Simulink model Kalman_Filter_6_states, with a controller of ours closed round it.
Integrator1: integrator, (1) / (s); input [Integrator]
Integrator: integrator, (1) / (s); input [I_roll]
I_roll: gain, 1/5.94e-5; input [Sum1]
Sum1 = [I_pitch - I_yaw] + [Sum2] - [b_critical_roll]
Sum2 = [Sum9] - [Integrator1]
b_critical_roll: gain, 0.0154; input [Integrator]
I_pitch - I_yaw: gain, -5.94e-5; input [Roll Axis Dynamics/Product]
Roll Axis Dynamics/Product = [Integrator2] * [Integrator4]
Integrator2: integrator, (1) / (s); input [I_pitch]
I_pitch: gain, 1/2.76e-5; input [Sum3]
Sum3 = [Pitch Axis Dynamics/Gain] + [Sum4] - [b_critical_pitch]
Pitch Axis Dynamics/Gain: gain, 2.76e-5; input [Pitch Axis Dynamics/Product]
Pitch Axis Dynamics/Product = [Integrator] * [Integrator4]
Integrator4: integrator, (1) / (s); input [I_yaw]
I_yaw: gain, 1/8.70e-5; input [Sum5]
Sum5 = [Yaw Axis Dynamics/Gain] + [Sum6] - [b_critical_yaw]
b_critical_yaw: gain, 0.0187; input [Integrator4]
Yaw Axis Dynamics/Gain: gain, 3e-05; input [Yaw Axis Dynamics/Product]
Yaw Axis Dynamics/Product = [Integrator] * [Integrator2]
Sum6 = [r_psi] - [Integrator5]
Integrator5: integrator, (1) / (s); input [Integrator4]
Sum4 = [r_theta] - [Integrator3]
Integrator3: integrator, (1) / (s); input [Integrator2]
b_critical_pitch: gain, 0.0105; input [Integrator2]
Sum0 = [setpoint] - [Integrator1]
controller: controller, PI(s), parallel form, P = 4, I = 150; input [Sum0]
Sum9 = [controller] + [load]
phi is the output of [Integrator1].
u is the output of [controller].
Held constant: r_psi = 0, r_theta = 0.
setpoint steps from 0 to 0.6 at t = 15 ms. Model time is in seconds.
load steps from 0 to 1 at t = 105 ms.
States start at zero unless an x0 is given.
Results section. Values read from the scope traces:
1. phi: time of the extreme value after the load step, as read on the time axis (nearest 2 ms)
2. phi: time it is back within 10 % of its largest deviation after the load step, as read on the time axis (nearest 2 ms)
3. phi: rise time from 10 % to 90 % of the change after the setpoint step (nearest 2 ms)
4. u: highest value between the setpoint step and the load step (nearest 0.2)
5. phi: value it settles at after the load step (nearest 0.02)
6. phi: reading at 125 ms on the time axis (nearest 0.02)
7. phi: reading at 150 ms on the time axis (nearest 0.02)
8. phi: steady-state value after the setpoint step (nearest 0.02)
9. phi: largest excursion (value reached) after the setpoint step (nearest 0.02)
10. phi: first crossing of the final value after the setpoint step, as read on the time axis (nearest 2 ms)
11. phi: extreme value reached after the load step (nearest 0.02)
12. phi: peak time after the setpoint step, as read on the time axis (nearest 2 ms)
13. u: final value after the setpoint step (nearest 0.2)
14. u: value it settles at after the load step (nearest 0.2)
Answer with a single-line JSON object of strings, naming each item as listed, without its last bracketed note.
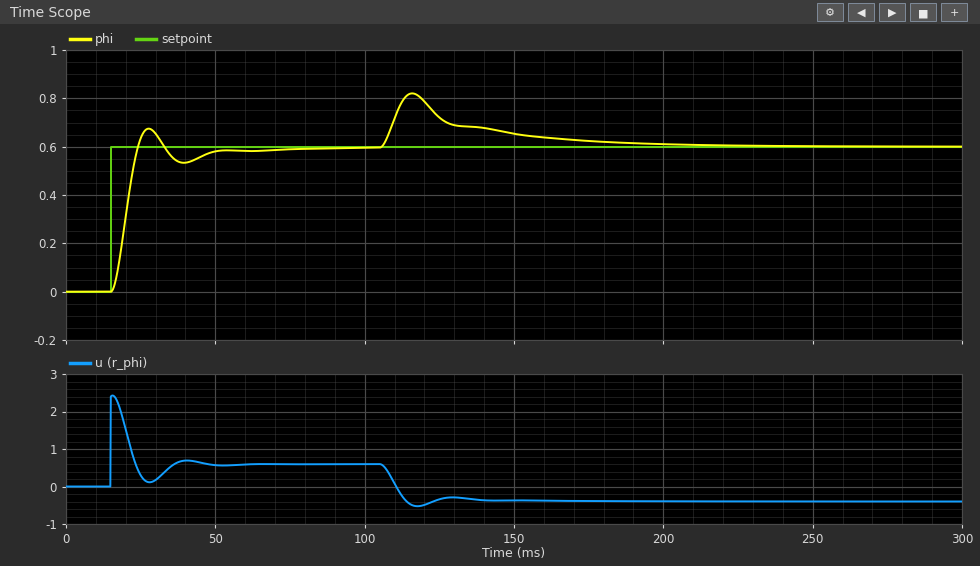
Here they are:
{"phi: time of the extreme value after the load step, as read on the time axis": "116 ms", "phi: time it is back within 10 % of its largest deviation after the load step, as read on the time axis": "176 ms", "phi: rise time from 10 % to 90 % of the change after the setpoint step": "6 ms", "u: highest value between the setpoint step and the load step": "2.4", "phi: value it settles at after the load step": "0.60", "phi: reading at 125 ms on the time axis": "0.72", "phi: reading at 150 ms on the time axis": "0.66", "phi: steady-state value after the setpoint step": "0.60", "phi: largest excursion (value reached) after the setpoint step": "0.68", "phi: first crossing of the final value after the setpoint step, as read on the time axis": "24 ms", "phi: extreme value reached after the load step": "0.82", "phi: peak time after the setpoint step, as read on the time axis": "28 ms", "u: final value after the setpoint step": "0.6", "u: value it settles at after the load step": "-0.4"}
